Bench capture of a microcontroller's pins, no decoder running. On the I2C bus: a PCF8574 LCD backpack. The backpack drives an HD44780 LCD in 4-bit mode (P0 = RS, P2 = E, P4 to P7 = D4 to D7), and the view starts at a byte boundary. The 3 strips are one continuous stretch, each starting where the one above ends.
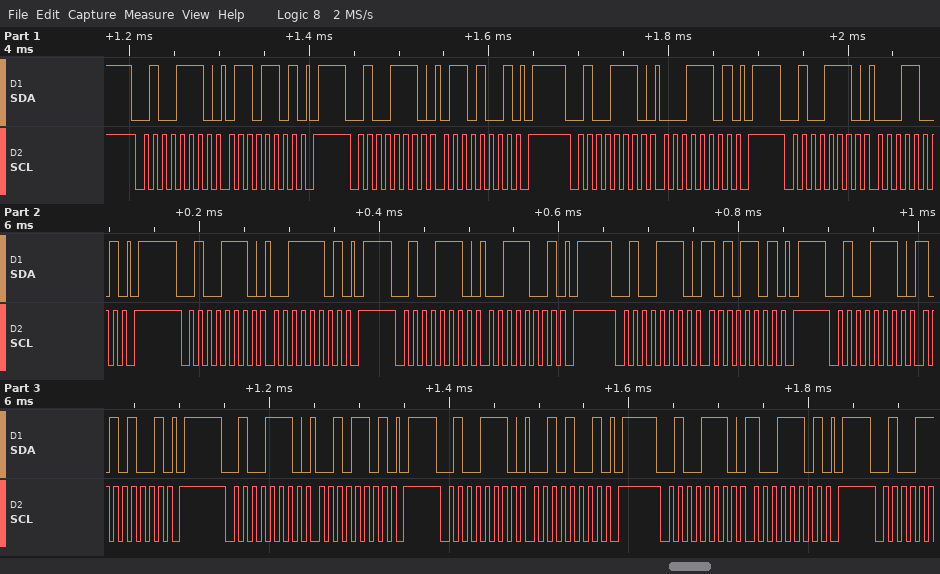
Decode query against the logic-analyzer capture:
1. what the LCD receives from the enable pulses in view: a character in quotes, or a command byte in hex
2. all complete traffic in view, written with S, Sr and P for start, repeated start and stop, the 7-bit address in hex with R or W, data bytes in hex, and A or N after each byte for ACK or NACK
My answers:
'a' ':'
S 27W A 6D A P S 27W A 69 A P S 27W A 1D A P S 27W A 19 A P S 27W A 3D A P S 27W A 39 A P S 27W A AD A P S 27W A A9 A P S 27W A 2D A P S 27W A 29 A P S 27W A 9D A P
